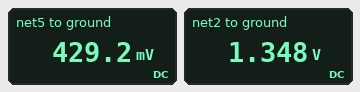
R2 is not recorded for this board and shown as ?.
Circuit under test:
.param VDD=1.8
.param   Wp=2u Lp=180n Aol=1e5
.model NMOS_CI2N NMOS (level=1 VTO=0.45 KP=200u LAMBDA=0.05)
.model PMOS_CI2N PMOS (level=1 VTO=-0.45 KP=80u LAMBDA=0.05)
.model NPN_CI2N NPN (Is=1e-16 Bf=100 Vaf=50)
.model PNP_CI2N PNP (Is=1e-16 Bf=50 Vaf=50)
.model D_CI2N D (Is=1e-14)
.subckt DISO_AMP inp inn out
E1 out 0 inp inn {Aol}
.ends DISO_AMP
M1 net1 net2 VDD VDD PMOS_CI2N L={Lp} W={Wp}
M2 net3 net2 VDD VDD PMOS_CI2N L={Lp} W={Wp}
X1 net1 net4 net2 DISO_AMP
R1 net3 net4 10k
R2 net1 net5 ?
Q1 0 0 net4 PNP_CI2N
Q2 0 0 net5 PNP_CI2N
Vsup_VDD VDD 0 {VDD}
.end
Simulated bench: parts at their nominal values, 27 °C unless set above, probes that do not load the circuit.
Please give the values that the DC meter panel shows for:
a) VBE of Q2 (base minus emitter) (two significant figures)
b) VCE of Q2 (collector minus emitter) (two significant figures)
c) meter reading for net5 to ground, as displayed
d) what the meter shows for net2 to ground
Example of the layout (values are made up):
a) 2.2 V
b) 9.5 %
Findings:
a) -430 mV
b) -430 mV
c) 429.2 mV
d) 1.348 V
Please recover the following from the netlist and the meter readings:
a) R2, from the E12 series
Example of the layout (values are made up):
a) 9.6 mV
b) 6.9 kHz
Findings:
a) 8.2 kΩ
